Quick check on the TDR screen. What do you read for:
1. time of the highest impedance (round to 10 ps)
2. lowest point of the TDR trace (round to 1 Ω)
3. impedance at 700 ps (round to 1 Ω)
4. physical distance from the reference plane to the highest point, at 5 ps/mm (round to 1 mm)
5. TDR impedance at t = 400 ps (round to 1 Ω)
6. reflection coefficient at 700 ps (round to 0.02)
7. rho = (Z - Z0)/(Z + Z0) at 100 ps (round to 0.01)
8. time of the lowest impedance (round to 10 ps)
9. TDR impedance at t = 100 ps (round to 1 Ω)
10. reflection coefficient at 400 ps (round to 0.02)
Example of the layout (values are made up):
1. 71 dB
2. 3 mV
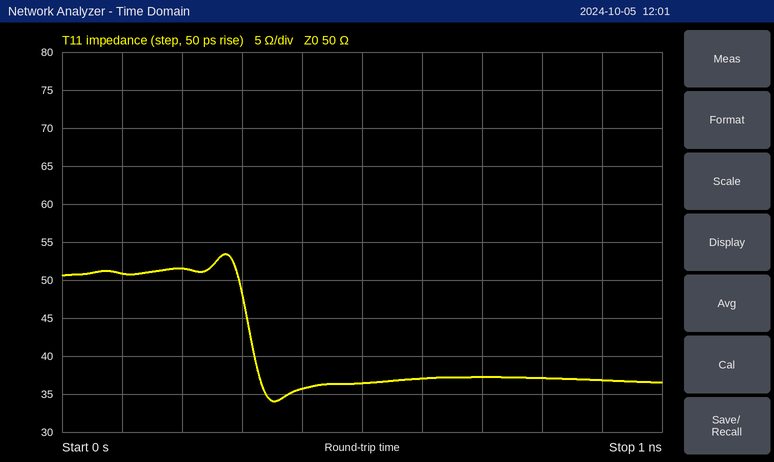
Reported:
1. 270 ps
2. 34 Ω
3. 37 Ω
4. 27 mm
5. 36 Ω
6. -0.14
7. +0.01
8. 350 ps
9. 51 Ω
10. -0.16
